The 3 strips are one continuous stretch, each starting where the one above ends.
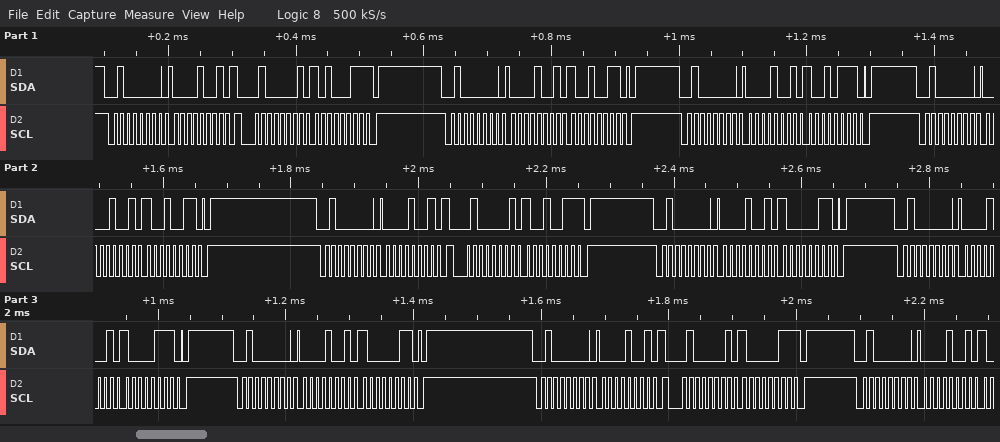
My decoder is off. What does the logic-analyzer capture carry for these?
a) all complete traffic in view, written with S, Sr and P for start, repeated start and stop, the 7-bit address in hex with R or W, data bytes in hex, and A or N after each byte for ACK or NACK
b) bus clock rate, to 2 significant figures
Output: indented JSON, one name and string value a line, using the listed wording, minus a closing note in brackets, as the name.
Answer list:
{
  "all complete traffic in view, written with S, Sr and P for start, repeated start and stop, the 7-bit address in hex with R or W, data bytes in hex, and A or N after each byte for ACK or NACK": "S 20W A 09 A Sr 20R A A3 N P S 20W A 09 A 93 A P S 20W A 09 A 97 A P S 20W A 09 A 93 A P S 20W A 09 A Sr 20R A 93 N P S 20W A 09 A 83 A P S 20W A 09 A 87 A P S 20W A 09 A 83 A P S 20W A 09 A Sr 20R A 83 N P S 20W A 09 A",
  "bus clock rate, to 2 significant figures": "100 kHz"
}
